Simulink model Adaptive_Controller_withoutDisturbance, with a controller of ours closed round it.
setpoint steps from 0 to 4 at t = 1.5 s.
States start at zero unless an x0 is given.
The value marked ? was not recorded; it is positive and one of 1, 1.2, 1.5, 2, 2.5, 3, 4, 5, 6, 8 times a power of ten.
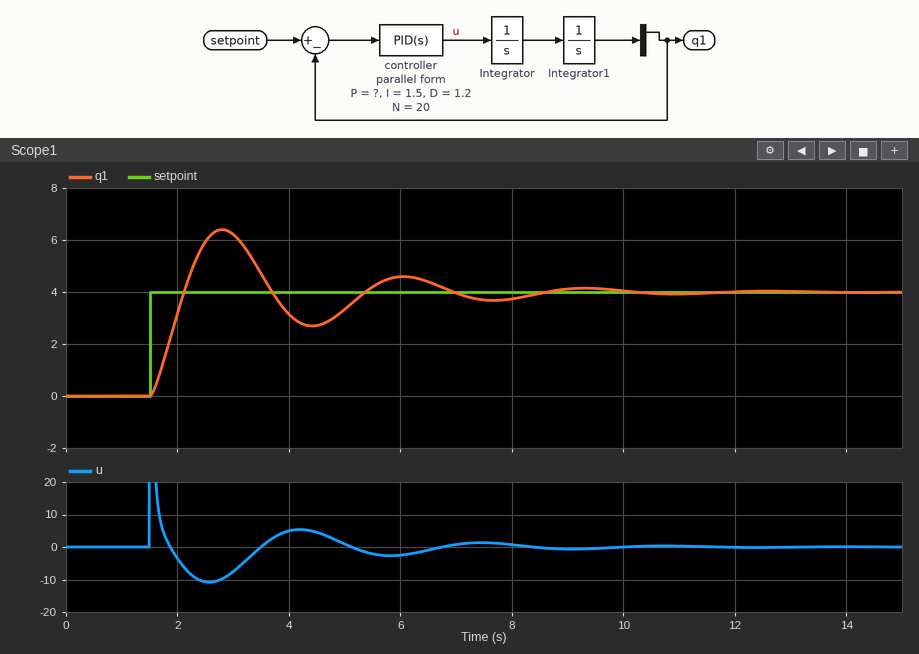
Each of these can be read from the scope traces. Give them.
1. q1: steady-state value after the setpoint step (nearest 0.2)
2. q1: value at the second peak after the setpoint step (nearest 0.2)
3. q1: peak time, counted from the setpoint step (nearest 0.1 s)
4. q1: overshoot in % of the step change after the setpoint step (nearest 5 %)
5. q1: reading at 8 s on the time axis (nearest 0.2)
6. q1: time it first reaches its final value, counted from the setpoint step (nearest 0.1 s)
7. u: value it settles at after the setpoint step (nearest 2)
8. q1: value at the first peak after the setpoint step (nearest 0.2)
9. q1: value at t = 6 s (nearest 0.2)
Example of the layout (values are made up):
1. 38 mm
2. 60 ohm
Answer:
1. 4.0
2. 4.6
3. 1.3 s
4. 60 %
5. 3.8
6. 0.6 s
7. 0
8. 6.4
9. 4.6
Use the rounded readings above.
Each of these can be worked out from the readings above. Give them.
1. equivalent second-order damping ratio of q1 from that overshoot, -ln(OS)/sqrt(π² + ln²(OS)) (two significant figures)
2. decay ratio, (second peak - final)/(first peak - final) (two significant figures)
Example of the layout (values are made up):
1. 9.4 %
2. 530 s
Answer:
1. 0.16
2. 0.25
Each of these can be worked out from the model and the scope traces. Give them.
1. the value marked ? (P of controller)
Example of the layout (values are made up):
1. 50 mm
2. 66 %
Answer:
1. 4
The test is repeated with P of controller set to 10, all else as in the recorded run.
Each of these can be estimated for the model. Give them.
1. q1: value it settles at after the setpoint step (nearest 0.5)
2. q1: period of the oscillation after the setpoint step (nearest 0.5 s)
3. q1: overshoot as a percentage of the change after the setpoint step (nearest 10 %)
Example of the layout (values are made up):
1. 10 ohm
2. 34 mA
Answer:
1. 4.0
2. 2.0 s
3. 70 %
